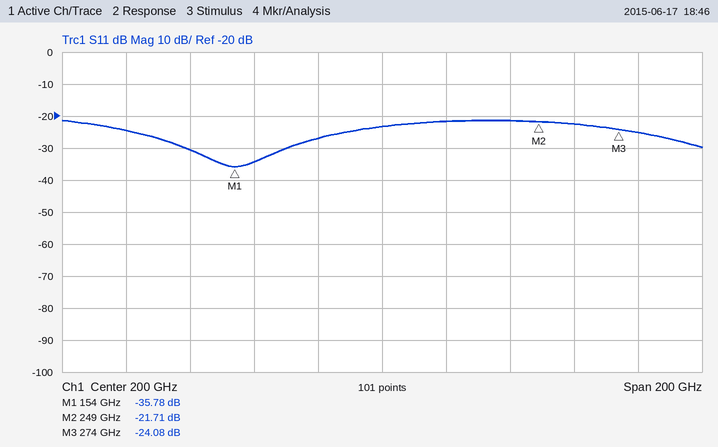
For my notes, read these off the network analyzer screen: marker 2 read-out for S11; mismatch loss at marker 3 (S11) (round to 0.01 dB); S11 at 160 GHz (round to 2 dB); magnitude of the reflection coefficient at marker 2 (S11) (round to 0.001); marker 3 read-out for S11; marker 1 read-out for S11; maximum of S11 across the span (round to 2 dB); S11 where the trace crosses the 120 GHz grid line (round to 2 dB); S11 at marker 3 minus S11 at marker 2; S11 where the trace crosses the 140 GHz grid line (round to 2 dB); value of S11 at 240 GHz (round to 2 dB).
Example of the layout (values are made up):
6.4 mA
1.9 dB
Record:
-21.71 dB
0.02 dB
-34 dB
0.082
-24.08 dB
-35.78 dB
-22 dB
-24 dB
-2.37 dB
-30 dB
-22 dB
